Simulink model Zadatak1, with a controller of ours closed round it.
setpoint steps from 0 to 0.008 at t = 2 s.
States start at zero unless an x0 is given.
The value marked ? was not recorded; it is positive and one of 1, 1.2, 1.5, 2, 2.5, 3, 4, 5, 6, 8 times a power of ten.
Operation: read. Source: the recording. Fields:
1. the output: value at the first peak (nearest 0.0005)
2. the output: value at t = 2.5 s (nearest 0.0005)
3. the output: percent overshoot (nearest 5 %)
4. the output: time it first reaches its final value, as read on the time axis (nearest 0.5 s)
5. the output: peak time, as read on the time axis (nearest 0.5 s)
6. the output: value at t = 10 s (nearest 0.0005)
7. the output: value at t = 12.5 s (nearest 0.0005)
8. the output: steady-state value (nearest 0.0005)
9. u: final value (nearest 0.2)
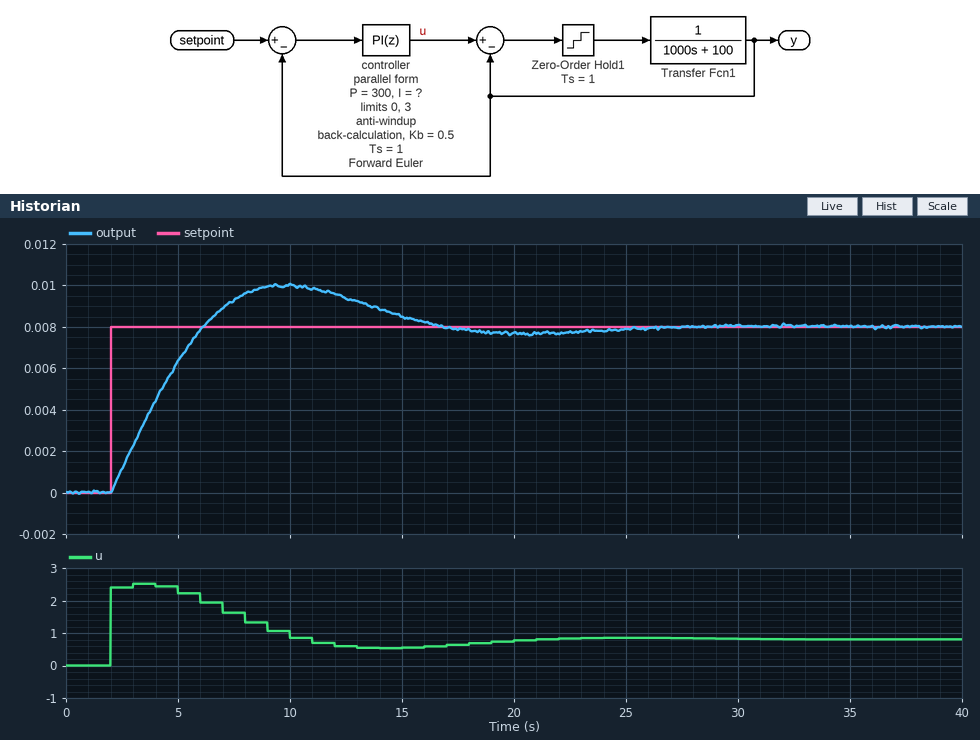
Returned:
0.0100
0.0010
25 %
6.0 s
10.0 s
0.0100
0.0095
0.0080
0.8
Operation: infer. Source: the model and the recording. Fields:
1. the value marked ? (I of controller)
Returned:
100
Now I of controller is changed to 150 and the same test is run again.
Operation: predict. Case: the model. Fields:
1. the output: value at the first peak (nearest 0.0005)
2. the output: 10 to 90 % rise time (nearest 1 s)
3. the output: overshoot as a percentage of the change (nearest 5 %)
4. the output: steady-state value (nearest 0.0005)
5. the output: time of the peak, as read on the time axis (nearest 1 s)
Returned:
0.0110
3 s
40 %
0.0080
9 s
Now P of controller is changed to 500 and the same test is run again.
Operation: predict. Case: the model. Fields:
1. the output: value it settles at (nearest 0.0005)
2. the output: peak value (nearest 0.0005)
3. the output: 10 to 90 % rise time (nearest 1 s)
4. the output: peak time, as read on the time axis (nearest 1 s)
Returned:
0.0080
0.0085
3 s
9 s
